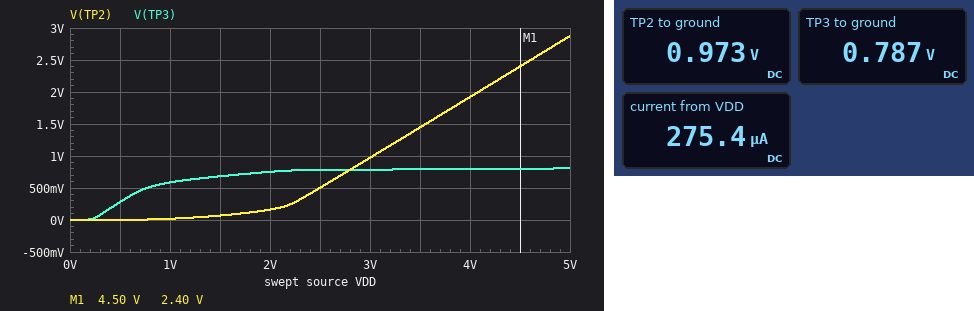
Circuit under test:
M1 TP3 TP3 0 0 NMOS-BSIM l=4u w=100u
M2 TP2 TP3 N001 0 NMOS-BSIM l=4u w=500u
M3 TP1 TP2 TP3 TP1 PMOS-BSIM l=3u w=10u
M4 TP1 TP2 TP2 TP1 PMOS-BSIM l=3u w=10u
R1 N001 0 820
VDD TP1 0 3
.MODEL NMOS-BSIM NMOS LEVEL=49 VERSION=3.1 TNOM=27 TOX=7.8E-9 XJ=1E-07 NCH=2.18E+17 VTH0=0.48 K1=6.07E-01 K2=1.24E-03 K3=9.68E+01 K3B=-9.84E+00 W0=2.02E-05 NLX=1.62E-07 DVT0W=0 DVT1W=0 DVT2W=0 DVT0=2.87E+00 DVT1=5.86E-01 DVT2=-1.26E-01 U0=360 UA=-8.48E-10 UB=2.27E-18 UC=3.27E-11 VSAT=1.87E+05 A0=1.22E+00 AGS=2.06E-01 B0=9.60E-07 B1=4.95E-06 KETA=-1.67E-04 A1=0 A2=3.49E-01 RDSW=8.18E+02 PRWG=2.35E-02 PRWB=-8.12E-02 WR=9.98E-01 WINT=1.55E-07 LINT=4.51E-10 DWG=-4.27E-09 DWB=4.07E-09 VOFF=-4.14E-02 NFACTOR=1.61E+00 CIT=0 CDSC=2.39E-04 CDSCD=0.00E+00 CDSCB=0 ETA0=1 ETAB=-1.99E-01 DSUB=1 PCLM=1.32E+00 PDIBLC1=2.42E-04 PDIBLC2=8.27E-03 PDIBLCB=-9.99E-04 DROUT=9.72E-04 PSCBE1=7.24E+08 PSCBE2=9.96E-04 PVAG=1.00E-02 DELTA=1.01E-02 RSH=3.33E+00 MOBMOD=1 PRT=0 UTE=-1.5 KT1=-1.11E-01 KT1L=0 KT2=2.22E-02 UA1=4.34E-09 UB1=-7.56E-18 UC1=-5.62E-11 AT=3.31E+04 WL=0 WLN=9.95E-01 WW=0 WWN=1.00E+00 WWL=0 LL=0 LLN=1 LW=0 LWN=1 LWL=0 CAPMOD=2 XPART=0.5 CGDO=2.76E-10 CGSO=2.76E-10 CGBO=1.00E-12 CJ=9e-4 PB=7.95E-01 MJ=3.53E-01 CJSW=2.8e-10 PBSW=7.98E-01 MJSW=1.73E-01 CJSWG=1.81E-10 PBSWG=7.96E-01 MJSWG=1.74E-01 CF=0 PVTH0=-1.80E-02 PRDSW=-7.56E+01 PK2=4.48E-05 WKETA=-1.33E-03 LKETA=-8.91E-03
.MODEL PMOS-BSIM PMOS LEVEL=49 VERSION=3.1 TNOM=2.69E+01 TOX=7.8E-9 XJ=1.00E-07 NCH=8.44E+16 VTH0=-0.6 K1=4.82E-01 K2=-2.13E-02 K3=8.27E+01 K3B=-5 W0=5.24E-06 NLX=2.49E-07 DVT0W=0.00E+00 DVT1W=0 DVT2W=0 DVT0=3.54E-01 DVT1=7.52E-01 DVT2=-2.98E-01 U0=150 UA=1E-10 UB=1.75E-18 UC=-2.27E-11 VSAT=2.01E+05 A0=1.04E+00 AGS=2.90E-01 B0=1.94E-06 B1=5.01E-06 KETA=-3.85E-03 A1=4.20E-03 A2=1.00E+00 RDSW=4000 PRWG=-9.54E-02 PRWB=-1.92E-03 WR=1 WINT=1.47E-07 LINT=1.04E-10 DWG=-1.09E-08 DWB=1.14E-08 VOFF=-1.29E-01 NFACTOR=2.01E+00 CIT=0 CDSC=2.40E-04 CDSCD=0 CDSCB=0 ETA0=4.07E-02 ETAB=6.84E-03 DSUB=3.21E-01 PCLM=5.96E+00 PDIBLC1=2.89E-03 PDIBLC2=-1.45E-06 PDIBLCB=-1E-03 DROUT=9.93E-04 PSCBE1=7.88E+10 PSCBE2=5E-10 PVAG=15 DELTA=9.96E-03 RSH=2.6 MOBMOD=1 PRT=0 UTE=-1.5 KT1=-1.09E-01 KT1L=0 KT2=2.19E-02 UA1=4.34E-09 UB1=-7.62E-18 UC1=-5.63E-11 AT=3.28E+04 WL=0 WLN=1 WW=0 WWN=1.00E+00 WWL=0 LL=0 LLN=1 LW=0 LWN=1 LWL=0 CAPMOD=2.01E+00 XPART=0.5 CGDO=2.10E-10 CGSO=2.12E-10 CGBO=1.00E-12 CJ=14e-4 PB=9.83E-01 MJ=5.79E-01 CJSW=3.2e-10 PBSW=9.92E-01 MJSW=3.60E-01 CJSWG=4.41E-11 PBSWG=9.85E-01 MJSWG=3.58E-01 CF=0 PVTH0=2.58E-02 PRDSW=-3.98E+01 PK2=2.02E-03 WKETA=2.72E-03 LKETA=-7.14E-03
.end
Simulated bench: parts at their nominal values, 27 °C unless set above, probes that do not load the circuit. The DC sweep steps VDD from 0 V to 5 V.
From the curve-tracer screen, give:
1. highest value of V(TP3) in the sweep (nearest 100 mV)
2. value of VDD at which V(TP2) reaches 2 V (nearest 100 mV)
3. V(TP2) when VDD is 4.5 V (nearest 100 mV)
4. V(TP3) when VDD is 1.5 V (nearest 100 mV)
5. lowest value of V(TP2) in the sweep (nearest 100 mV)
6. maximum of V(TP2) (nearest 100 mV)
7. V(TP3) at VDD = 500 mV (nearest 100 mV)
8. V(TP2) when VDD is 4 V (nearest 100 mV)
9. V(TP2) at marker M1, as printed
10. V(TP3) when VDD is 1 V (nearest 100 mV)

800 mV
4.1 V
2.4 V
700 mV
0 V
2.9 V
300 mV
1.9 V
2.40 V
600 mV
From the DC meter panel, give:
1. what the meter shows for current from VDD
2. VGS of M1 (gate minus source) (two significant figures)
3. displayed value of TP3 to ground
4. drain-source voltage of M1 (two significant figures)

275.4 µA
790 mV
0.787 V
790 mV
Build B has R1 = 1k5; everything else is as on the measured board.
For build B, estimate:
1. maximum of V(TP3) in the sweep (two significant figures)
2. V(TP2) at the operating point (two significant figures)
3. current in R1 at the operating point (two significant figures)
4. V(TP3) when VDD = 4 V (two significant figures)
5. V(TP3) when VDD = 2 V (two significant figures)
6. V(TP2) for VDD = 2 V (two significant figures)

710 mV
1.5 V
56 µA
700 mV
690 mV
530 mV
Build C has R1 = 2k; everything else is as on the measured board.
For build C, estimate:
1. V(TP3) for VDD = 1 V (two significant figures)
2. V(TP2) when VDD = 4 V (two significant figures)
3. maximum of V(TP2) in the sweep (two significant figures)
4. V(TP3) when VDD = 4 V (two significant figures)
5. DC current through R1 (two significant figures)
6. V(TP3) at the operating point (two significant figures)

580 mV
2.6 V
3.6 V
680 mV
39 µA
670 mV
